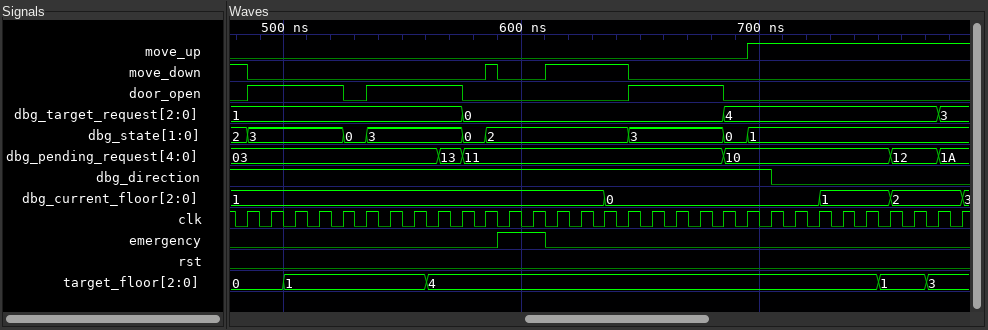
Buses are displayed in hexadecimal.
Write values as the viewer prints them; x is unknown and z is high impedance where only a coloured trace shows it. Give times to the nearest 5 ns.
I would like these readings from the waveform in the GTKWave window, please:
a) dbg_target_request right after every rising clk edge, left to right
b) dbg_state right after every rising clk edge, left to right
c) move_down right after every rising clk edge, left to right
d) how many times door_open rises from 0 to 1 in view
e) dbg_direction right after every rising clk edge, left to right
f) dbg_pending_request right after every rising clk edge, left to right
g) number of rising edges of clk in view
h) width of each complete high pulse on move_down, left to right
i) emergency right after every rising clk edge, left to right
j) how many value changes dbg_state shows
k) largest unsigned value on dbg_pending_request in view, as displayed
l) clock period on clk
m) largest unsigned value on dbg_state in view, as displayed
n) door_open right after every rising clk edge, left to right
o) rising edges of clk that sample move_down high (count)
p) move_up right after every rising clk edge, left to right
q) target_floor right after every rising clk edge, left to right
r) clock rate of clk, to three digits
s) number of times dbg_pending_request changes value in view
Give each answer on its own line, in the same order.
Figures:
1, 1, 1, 1, 1, 1, 1, 1, 1, 0, 0, 0, 0, 0, 0, 0, 0, 0, 0, 0, 4, 4, 4, 4, 4, 4, 4, 4, 4, 3, 3
3, 3, 3, 3, 0, 3, 3, 3, 3, 0, 2, 2, 2, 2, 2, 2, 3, 3, 3, 3, 0, 1, 1, 1, 1, 1, 1, 1, 1, 1, 1
0 0 0 0 0 0 0 0 0 0 1 0 0 1 1 1 0 0 0 0 0 0 0 0 0 0 0 0 0 0 0
3
1 1 1 1 1 1 1 1 1 1 1 1 1 1 1 1 1 1 1 1 1 1 0 0 0 0 0 0 0 0 0
03, 03, 03, 03, 03, 03, 03, 03, 13, 11, 11, 11, 11, 11, 11, 11, 11, 11, 11, 11, 10, 10, 10, 10, 10, 10, 10, 12, 12, 1A, 1A
31
5 ns, 35 ns
0 0 0 0 0 0 0 0 0 0 0 1 1 0 0 0 0 0 0 0 0 0 0 0 0 0 0 0 0 0 0
8
1A
10 ns
3
1 1 1 1 0 1 1 1 1 0 0 0 0 0 0 0 1 1 1 1 0 0 0 0 0 0 0 0 0 0 0
5
0 0 0 0 0 0 0 0 0 0 0 0 0 0 0 0 0 0 0 0 0 1 1 1 1 1 1 1 1 1 1
0, 0, 1, 1, 1, 1, 1, 1, 4, 4, 4, 4, 4, 4, 4, 4, 4, 4, 4, 4, 4, 4, 4, 4, 4, 4, 4, 1, 1, 3, 3
100 MHz
5
